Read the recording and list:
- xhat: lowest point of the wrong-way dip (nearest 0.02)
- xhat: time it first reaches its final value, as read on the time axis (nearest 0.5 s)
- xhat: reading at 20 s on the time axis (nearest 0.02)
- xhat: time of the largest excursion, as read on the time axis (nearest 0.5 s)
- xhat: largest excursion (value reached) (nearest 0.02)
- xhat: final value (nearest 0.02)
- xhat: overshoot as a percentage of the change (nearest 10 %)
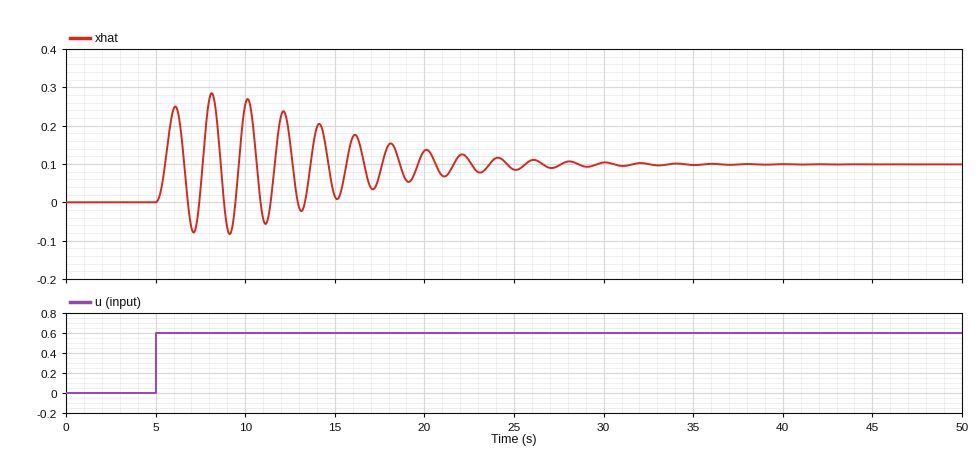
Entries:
-0.08
5.5 s
0.14
8.0 s
0.28
0.10
190 %
